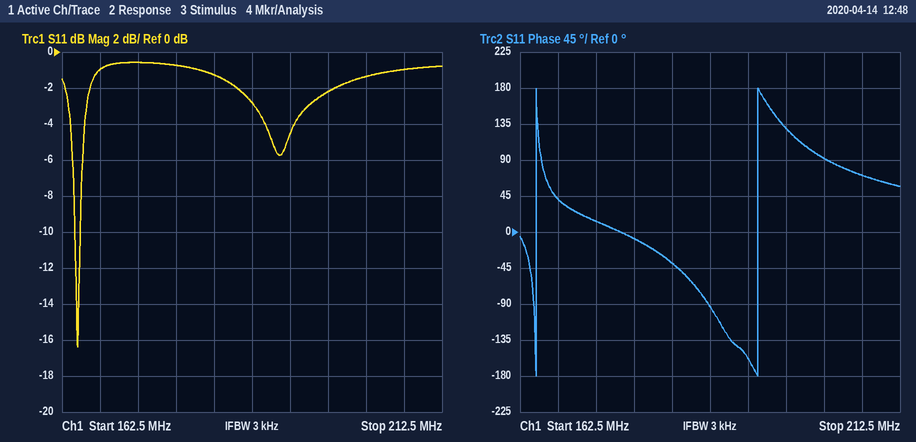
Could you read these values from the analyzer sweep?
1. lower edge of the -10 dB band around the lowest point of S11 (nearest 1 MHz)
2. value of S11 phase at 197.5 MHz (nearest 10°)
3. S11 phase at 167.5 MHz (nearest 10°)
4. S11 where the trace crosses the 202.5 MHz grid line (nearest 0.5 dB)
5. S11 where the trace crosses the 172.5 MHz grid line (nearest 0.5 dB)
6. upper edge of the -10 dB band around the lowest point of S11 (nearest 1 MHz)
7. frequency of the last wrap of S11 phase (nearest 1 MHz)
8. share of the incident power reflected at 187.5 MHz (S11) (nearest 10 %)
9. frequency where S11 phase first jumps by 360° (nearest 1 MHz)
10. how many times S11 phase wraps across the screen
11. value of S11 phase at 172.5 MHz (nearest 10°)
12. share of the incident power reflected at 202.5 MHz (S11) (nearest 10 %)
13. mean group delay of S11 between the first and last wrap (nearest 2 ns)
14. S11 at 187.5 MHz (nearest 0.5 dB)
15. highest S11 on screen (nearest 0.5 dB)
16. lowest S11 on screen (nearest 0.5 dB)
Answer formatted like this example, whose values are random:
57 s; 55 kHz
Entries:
164 MHz; 130°; 40°; -1.5 dB; -0.5 dB; 165 MHz; 194 MHz; 50 %; 165 MHz; 2; 10°; 70 %; 34 ns; -3.0 dB; -0.5 dB; -16.5 dB
